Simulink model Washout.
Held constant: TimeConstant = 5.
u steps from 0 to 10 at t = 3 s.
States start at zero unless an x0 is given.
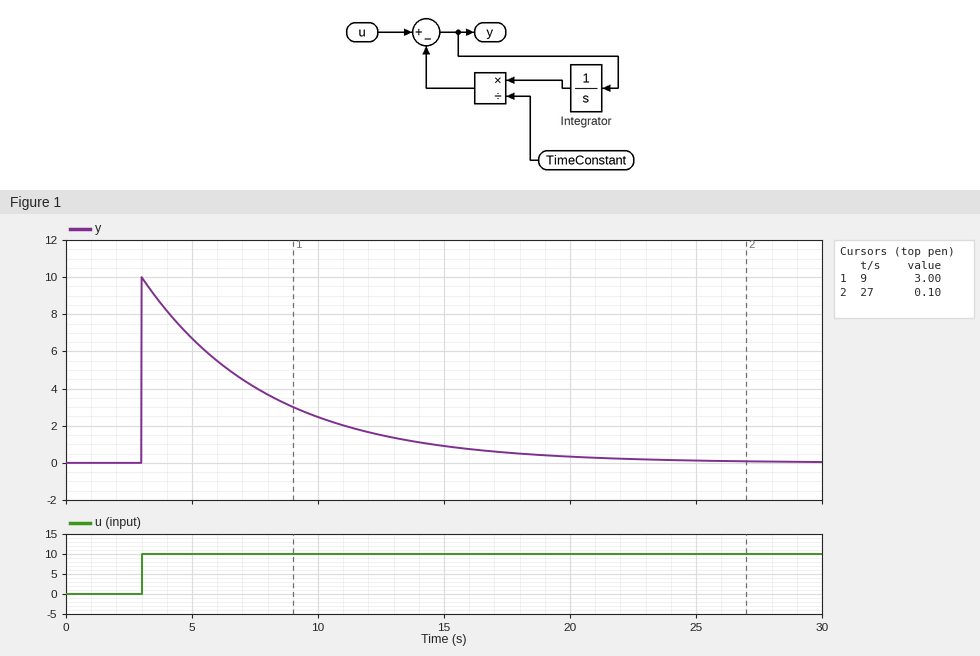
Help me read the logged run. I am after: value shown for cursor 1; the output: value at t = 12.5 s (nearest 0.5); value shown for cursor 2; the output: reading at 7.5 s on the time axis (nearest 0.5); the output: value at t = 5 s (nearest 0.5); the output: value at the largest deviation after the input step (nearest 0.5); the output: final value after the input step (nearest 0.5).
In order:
3.00
1.5
0.10
4.0
6.5
10.0
0.0
